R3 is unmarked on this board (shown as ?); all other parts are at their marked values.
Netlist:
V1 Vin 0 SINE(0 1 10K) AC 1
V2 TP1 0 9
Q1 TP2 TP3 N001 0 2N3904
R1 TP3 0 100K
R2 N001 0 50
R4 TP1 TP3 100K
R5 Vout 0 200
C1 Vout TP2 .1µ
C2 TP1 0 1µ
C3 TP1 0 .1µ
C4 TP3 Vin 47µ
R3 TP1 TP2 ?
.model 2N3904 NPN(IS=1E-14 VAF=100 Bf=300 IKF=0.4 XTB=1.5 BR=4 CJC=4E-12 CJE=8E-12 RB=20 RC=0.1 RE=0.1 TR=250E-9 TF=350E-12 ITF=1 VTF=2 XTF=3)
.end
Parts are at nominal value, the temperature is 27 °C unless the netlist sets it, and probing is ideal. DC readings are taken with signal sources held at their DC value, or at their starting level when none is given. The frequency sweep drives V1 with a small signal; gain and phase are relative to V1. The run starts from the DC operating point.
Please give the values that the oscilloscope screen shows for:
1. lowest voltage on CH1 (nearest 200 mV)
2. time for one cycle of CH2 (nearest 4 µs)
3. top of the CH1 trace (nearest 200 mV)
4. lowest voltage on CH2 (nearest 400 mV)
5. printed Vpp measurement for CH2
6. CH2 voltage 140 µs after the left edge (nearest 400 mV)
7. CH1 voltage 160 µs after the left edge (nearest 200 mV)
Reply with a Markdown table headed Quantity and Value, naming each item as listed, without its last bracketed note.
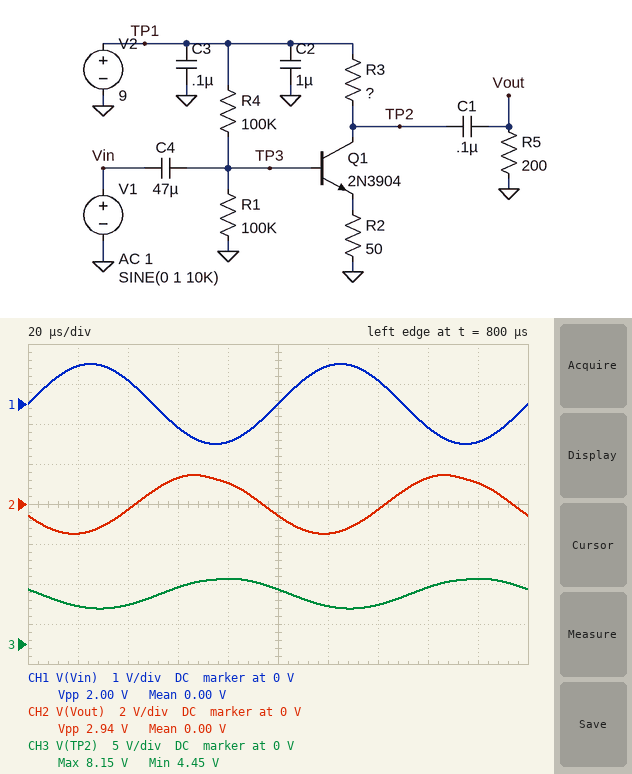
| Quantity | Value |
|---|---|
| lowest voltage on CH1 | -1.0 V |
| time for one cycle of CH2 | 100 µs |
| top of the CH1 trace | 1.0 V |
| lowest voltage on CH2 | -1.6 V |
| printed Vpp measurement for CH2 | 2.94 V |
| CH2 voltage 140 µs after the left edge | -400 mV |
| CH1 voltage 160 µs after the left edge | -600 mV |
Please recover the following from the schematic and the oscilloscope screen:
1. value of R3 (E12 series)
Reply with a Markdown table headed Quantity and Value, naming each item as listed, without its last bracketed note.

| Quantity | Value |
|---|---|
| value of R3 | 150 Ω |
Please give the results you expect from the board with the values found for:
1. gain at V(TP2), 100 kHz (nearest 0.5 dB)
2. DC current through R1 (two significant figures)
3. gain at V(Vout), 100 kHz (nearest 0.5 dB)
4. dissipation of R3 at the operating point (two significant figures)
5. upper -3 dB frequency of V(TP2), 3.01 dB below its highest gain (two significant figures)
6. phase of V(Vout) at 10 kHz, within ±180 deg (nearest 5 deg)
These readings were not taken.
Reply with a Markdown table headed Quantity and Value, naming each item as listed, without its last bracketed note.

| Quantity | Value |
|---|---|
| gain at V(TP2), 100 kHz | 4.5 dB |
| DC current through R1 | 16 µA |
| gain at V(Vout), 100 kHz | 4.5 dB |
| dissipation of R3 at the operating point | 46 mW |
| upper -3 dB frequency of V(TP2), 3.01 dB below its highest gain | 7.7 kHz |
| phase of V(Vout) at 10 kHz, within ±180 deg | -155 deg |
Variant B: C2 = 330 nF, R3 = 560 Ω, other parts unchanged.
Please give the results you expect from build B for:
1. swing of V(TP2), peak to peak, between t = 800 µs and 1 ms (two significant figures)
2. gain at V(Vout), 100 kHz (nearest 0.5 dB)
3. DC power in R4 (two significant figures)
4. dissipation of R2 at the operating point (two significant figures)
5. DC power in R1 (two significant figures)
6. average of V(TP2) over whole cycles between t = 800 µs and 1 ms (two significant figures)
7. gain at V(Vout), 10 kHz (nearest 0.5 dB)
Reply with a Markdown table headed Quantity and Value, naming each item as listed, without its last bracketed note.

| Quantity | Value |
|---|---|
| swing of V(TP2), peak to peak, between t = 800 µs and 1 ms | 4.3 V |
| gain at V(Vout), 100 kHz | 8.0 dB |
| DC power in R4 | 570 µW |
| dissipation of R2 at the operating point | 11 mW |
| DC power in R1 | 21 µW |
| average of V(TP2) over whole cycles between t = 800 µs and 1 ms | 2.8 V |
| gain at V(Vout), 10 kHz | 7.5 dB |
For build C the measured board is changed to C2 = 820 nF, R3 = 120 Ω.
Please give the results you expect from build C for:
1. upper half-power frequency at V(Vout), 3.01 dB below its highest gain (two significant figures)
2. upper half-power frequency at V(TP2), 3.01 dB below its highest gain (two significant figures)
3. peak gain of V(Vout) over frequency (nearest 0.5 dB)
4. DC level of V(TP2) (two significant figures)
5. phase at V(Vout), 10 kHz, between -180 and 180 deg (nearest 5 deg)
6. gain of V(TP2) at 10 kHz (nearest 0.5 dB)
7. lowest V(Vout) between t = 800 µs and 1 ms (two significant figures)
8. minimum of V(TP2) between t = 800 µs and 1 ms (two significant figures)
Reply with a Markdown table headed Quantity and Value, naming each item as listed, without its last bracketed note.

| Quantity | Value |
|---|---|
| upper half-power frequency at V(Vout), 3.01 dB below its highest gain | 330 MHz |
| upper half-power frequency at V(TP2), 3.01 dB below its highest gain | 11 kHz |
| peak gain of V(Vout) over frequency | 3.0 dB |
| DC level of V(TP2) | 6.9 V |
| phase at V(Vout), 10 kHz, between -180 and 180 deg | -155 deg |
| gain of V(TP2) at 10 kHz | 4.5 dB |
| lowest V(Vout) between t = 800 µs and 1 ms | -1.3 V |
| minimum of V(TP2) between t = 800 µs and 1 ms | 5.2 V |
